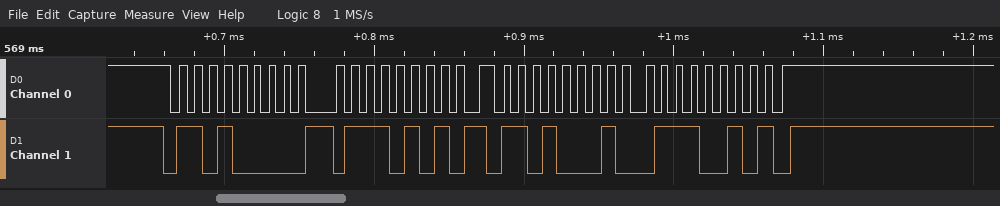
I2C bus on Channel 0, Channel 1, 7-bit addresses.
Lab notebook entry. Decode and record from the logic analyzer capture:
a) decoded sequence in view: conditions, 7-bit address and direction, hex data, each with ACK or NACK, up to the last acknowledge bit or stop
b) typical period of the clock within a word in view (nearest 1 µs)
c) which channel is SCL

start, address 68 write ACK, 75 ACK, repeated start, address 68 read ACK, 72 NACK, stop
10 µs
Channel 0
